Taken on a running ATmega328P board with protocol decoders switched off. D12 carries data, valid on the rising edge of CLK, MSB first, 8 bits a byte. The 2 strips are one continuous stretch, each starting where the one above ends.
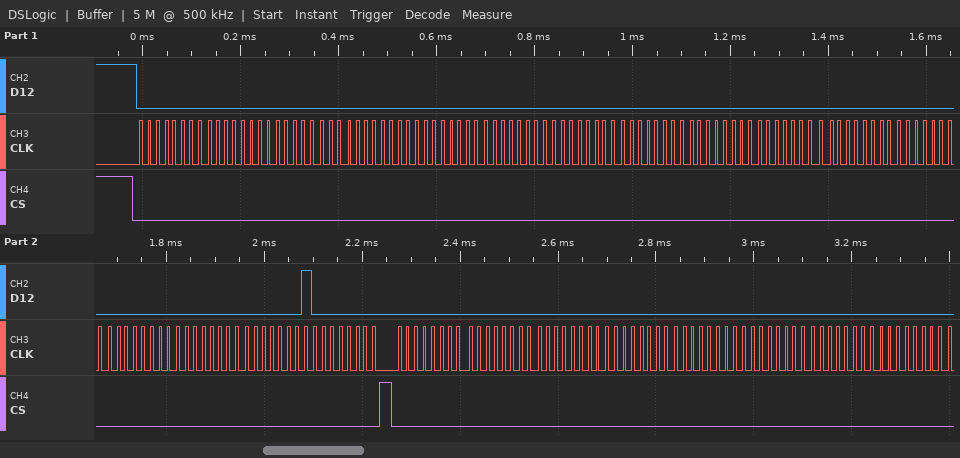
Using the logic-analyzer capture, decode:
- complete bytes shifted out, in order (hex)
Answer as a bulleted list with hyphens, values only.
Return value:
- 00 00 00 00 00 00 00 00 00 00 00 00 00 00 01 00 00 00 00 00 00 00 00 00
